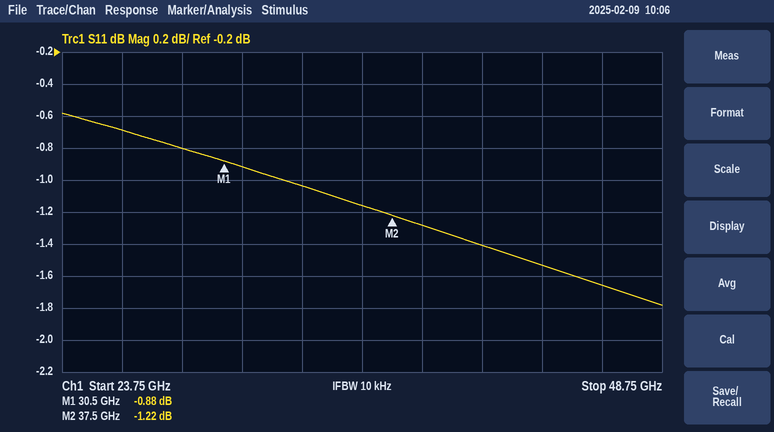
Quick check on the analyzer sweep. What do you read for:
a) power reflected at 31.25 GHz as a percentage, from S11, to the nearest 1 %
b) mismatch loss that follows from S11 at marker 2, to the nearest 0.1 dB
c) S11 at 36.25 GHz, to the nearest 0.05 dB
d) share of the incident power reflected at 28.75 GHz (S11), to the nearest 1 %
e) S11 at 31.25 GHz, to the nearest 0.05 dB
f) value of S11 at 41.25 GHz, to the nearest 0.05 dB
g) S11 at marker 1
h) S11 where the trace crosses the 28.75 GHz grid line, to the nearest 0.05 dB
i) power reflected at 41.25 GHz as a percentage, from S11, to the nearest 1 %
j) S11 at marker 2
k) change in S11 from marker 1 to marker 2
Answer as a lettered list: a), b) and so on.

a) 81 %
b) 6.1 dB
c) -1.15 dB
d) 83 %
e) -0.90 dB
f) -1.40 dB
g) -0.88 dB
h) -0.80 dB
i) 72 %
j) -1.22 dB
k) -0.34 dB
